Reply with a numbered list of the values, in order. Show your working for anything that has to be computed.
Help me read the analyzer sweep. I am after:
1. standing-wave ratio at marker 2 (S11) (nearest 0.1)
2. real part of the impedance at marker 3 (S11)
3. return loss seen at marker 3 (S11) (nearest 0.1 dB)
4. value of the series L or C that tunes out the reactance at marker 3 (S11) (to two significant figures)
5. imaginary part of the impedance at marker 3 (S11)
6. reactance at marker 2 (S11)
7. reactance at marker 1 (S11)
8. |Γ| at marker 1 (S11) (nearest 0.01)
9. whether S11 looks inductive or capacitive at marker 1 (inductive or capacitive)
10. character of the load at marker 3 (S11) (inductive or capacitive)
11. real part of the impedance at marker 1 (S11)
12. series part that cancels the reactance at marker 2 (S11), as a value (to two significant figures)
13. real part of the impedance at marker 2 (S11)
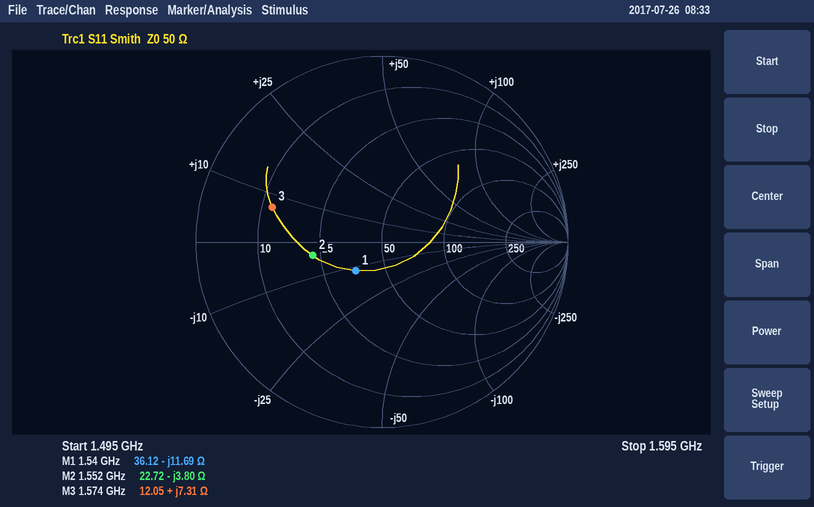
1. 2.2
2. 12.05 Ω
3. 4.2 dB
4. C = 1/(2π × 1.574 GHz × 7.31 Ω) ≈ 14 pF
5. +7.31 Ω
6. -3.80 Ω
7. -11.69 Ω
8. 0.21
9. capacitive
10. inductive
11. 36.12 Ω
12. L = 3.8 Ω/(2π × 1.552 GHz) ≈ 390 pH
13. 22.72 Ω
